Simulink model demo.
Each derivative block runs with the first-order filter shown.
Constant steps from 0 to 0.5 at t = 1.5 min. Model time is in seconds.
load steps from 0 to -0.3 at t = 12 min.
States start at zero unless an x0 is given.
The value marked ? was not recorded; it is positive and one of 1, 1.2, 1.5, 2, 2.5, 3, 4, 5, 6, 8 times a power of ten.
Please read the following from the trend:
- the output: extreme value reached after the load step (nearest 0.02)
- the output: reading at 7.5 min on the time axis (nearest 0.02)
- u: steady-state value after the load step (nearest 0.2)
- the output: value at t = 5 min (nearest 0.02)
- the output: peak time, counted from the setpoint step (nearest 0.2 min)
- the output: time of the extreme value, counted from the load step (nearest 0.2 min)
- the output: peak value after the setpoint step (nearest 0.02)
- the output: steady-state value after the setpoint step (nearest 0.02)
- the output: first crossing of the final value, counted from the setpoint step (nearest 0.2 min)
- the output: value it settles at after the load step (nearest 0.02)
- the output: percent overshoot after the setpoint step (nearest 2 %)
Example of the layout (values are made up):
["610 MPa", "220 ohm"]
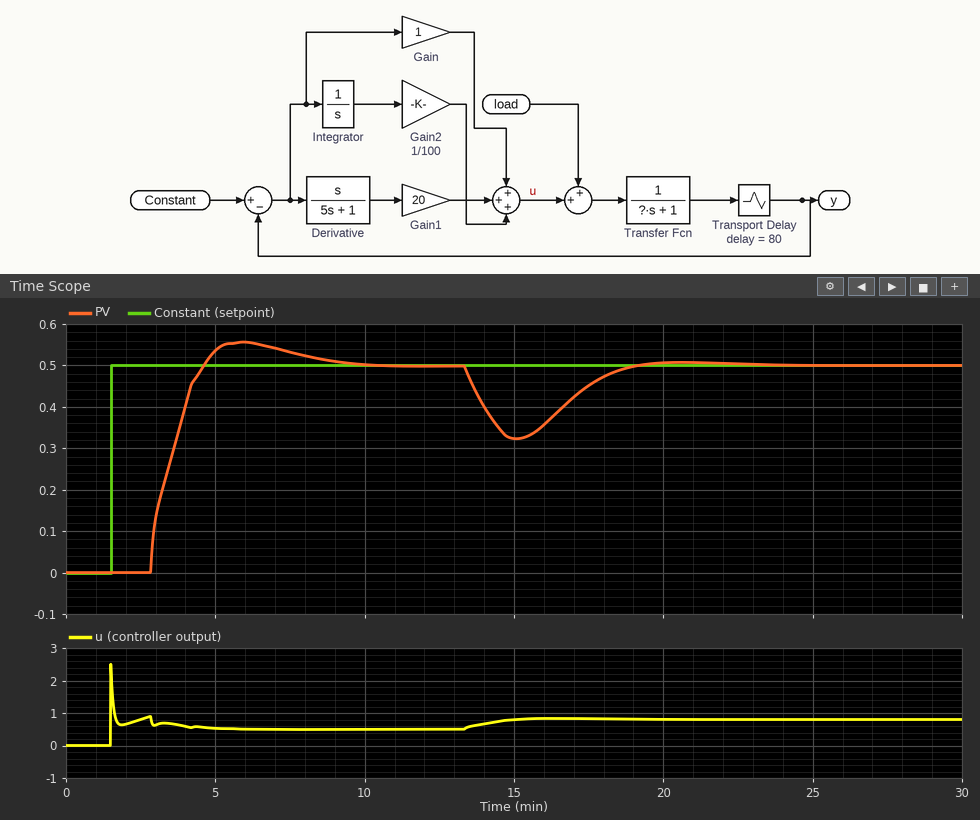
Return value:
["0.32", "0.54", "0.8", "0.54", "4.4 min", "3.0 min", "0.56", "0.50", "3.2 min", "0.50", "12 %"]
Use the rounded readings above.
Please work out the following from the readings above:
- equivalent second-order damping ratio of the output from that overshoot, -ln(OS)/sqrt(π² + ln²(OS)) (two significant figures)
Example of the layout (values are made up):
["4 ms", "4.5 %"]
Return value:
["0.56"]
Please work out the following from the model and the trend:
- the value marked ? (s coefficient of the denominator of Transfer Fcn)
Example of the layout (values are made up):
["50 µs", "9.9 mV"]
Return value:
["100"]
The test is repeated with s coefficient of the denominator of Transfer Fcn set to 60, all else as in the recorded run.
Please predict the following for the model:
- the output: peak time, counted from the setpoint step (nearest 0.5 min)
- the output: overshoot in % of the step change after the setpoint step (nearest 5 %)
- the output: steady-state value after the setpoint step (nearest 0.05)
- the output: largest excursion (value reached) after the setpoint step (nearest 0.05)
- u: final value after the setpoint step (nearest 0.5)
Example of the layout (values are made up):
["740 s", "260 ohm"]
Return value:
["2.5 min", "20 %", "0.50", "0.60", "0.5"]
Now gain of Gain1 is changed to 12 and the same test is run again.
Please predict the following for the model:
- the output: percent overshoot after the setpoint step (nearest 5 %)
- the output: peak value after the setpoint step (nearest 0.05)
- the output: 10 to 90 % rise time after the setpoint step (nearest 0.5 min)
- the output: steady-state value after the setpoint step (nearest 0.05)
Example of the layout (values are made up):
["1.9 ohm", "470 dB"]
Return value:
["20 %", "0.60", "1.5 min", "0.50"]
